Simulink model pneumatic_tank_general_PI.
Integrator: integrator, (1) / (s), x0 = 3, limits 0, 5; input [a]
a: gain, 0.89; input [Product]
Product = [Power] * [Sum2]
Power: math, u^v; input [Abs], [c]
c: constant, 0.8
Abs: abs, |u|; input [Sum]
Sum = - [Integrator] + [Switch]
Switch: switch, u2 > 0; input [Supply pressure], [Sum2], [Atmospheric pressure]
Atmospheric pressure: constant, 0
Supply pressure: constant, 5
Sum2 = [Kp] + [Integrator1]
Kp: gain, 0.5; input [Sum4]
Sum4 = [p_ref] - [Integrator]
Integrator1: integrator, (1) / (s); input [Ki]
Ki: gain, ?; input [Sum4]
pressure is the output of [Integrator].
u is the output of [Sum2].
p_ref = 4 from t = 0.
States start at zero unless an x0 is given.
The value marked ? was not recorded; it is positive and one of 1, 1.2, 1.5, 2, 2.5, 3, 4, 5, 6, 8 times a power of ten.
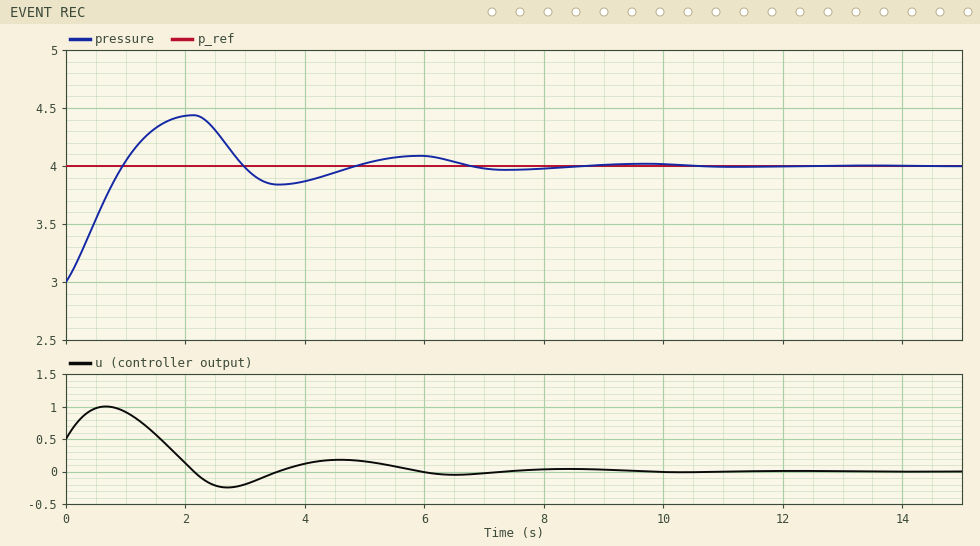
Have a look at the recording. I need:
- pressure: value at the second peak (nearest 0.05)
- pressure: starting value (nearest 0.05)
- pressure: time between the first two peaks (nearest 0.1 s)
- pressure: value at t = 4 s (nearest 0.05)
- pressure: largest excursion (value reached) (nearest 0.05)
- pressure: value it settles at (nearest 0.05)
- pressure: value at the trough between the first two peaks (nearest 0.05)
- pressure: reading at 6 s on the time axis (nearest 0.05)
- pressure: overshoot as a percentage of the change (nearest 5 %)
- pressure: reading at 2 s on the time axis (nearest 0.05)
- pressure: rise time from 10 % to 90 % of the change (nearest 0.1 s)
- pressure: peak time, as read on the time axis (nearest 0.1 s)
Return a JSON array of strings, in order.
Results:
["4.10", "3.00", "3.8 s", "3.85", "4.45", "4.00", "3.85", "4.10", "45 %", "4.45", "0.7 s", "2.1 s"]
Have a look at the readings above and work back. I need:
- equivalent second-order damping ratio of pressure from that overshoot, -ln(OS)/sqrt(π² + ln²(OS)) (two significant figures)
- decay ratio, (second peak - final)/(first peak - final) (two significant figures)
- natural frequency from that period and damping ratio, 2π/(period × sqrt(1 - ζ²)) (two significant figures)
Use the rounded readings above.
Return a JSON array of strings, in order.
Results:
["0.25", "0.22", "1.7 rad/s"]
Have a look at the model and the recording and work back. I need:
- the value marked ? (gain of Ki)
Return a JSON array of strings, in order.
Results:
["2"]
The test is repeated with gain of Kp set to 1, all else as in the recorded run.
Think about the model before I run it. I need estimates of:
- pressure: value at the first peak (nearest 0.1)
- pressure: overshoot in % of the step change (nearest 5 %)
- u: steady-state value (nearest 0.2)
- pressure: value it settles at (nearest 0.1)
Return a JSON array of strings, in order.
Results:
["4.3", "30 %", "0.0", "4.0"]
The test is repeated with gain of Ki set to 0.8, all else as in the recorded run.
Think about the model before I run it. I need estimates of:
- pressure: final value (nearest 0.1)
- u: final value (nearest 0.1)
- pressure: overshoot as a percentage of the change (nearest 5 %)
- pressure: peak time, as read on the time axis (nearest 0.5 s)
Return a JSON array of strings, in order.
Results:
["4.0", "0.0", "35 %", "3.0 s"]
